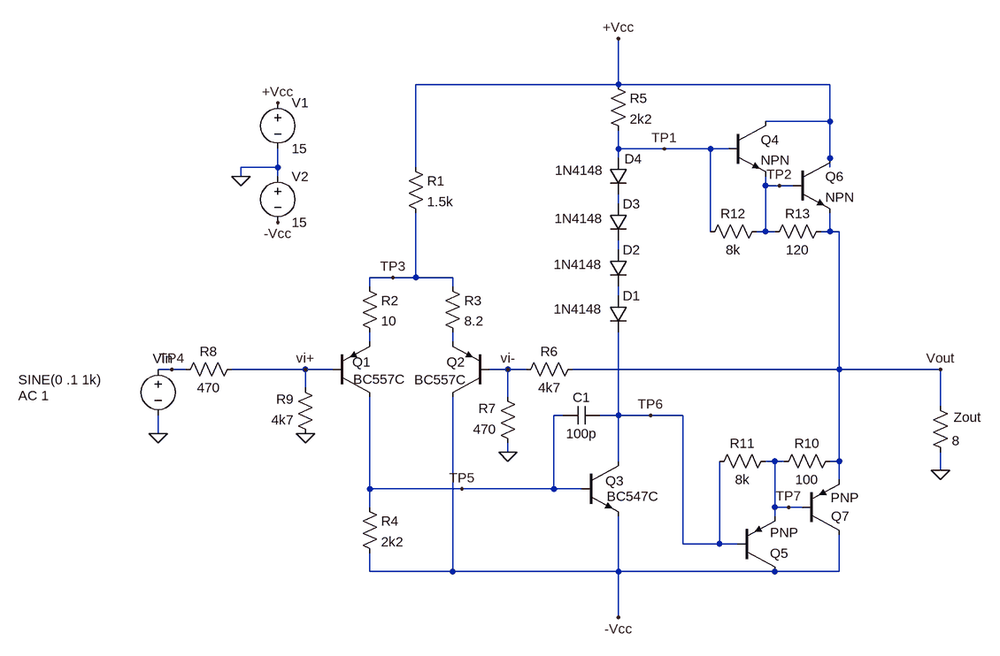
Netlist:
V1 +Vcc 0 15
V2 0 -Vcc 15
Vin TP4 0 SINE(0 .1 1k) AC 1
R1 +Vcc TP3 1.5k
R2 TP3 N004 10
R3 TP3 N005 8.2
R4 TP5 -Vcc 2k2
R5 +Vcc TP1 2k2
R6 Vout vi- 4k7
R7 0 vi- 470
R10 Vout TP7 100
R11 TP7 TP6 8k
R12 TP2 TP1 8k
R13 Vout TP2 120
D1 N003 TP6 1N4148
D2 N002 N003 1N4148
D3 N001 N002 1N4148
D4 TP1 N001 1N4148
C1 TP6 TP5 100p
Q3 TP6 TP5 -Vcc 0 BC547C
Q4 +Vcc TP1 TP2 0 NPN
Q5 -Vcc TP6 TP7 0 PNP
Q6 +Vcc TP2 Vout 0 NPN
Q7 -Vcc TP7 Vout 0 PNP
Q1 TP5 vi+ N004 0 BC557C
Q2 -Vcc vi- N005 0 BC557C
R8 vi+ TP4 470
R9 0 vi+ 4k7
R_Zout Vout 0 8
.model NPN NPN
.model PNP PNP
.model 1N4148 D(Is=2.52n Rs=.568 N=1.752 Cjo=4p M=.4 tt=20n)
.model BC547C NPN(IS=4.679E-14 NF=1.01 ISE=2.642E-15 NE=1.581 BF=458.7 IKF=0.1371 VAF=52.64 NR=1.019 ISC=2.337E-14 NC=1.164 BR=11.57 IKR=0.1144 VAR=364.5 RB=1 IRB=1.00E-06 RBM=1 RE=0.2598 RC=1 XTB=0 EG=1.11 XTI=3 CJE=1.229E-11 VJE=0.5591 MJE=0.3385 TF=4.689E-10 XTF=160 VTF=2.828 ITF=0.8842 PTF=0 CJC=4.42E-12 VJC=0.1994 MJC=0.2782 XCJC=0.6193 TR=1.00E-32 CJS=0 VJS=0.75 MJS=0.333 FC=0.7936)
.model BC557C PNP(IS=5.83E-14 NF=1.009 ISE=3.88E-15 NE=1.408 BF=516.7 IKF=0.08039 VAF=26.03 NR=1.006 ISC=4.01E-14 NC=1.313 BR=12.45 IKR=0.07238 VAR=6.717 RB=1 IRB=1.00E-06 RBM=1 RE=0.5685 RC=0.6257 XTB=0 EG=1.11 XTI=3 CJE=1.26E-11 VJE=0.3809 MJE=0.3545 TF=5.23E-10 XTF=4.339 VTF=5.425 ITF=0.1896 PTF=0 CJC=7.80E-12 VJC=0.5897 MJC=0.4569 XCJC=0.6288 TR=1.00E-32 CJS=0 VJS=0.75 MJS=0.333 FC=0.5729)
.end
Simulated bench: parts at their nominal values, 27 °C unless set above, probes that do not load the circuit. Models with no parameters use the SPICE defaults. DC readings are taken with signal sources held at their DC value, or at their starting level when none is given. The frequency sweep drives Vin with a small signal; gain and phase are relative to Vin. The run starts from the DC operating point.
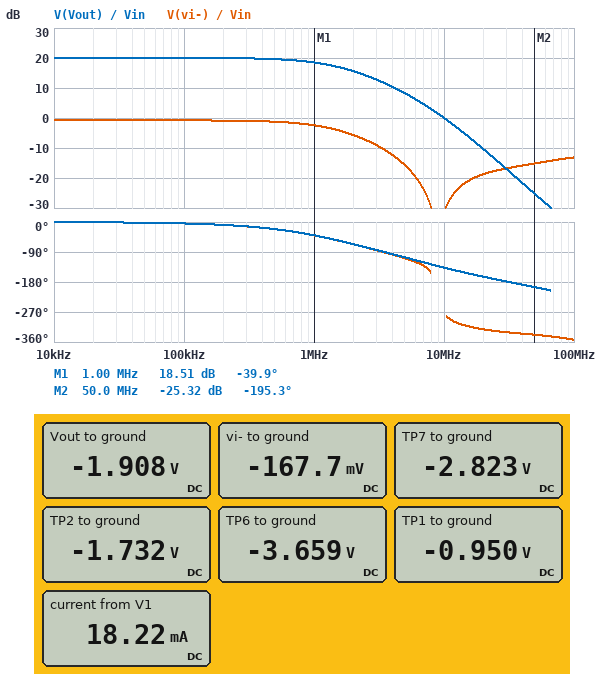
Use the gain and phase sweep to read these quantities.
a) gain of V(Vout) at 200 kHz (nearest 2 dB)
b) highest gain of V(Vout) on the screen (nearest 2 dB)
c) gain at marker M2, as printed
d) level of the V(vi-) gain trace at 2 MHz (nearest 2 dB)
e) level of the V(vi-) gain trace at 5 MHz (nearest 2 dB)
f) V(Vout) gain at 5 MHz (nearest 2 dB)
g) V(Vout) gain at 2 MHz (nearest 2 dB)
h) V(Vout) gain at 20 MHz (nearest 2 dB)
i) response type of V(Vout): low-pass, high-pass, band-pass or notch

20 dB
20 dB
-25.32 dB
-6 dB
-16 dB
8 dB
16 dB
-10 dB
low-pass
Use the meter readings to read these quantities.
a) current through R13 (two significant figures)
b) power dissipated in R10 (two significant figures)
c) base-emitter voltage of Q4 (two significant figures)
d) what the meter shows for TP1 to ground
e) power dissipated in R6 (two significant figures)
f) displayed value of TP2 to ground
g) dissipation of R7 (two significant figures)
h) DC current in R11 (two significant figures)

1.5 mA
8.4 mW
780 mV
-0.950 V
640 µW
-1.732 V
60 µW
100 µA
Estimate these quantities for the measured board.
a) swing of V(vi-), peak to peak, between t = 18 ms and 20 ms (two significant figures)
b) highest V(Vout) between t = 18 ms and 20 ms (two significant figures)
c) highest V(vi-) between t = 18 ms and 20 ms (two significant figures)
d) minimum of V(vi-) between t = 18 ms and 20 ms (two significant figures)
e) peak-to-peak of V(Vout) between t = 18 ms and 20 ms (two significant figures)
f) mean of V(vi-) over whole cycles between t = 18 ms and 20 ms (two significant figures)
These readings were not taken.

180 mV
-900 mV
-76 mV
-260 mV
2.0 V
-170 mV
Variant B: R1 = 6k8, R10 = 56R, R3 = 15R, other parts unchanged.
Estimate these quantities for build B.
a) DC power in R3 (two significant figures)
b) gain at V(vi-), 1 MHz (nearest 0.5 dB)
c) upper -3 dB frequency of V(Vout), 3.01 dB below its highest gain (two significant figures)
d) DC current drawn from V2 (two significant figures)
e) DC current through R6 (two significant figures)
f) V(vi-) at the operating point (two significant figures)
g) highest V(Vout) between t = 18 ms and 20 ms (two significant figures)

49 µW
-3.0 dB
1.2 MHz
110 mA
150 µA
-70 mV
220 mV
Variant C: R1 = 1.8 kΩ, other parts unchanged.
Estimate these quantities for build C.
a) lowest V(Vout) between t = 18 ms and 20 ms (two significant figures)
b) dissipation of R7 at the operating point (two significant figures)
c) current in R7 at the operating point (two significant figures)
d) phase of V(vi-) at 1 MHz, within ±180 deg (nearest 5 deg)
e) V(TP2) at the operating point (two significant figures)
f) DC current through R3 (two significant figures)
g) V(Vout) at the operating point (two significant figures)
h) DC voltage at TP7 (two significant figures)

-2.7 V
47 µW
320 µA
-40 deg
-1.5 V
7.7 mA
-1.7 V
-2.6 V
